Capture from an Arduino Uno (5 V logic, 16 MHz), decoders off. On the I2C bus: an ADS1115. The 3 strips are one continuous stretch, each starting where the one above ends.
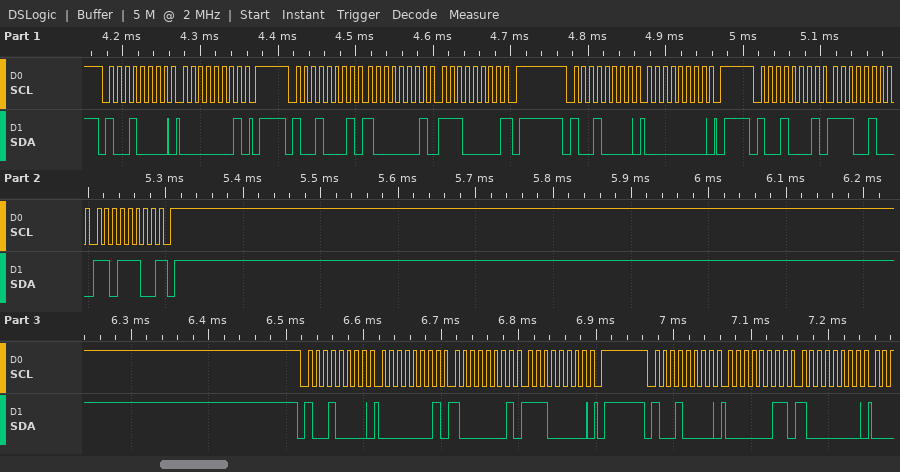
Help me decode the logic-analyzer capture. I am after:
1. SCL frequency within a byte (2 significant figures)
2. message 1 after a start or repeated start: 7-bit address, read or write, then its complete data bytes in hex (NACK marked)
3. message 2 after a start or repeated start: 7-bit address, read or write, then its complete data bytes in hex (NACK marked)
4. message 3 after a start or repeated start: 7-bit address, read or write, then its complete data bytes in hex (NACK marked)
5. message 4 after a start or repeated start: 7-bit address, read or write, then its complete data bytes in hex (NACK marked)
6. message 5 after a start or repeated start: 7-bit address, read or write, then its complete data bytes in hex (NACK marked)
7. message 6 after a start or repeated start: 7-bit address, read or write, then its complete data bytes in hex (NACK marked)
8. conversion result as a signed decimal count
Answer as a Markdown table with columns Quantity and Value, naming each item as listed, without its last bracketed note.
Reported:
| Quantity | Value |
|---|---|
| SCL frequency within a byte | 100 kHz |
| message 1 after a start or repeated start: 7-bit address, read or write, then its complete data bytes in hex | 0x48 write: 01 |
| message 2 after a start or repeated start: 7-bit address, read or write, then its complete data bytes in hex | 0x48 read: 81 E0 NACK |
| message 3 after a start or repeated start: 7-bit address, read or write, then its complete data bytes in hex | 0x48 write: 00 |
| message 4 after a start or repeated start: 7-bit address, read or write, then its complete data bytes in hex | 0x48 read: E4 DC NACK |
| message 5 after a start or repeated start: 7-bit address, read or write, then its complete data bytes in hex | 0x48 write: 01 81 E0 |
| message 6 after a start or repeated start: 7-bit address, read or write, then its complete data bytes in hex | 0x48 write: 03 80 |
| conversion result as a signed decimal count | -6948 |
